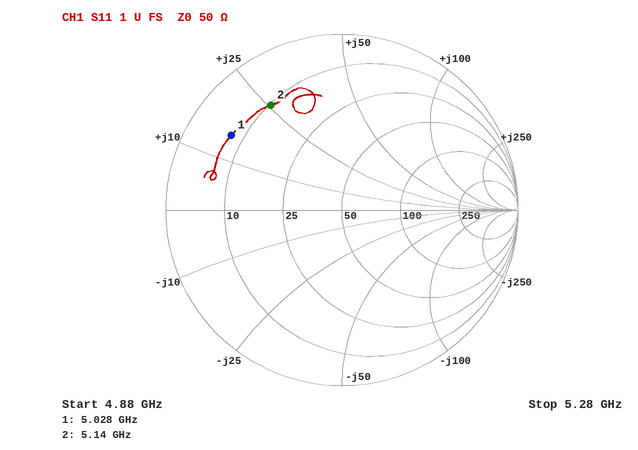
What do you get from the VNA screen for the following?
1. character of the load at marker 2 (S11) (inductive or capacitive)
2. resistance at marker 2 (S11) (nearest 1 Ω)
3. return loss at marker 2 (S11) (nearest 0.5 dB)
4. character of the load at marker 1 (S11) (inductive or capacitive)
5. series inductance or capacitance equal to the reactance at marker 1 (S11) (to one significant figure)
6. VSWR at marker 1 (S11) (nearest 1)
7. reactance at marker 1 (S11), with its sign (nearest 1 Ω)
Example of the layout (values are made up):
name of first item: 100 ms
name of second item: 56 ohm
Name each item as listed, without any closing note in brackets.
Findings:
character of the load at marker 2 (S11): inductive
resistance at marker 2 (S11): 10 Ω
return loss at marker 2 (S11): 3.0 dB
character of the load at marker 1 (S11): inductive
series inductance or capacitance equal to the reactance at marker 1 (S11): 500 pH
VSWR at marker 1 (S11): 7
reactance at marker 1 (S11), with its sign: +15 Ω
